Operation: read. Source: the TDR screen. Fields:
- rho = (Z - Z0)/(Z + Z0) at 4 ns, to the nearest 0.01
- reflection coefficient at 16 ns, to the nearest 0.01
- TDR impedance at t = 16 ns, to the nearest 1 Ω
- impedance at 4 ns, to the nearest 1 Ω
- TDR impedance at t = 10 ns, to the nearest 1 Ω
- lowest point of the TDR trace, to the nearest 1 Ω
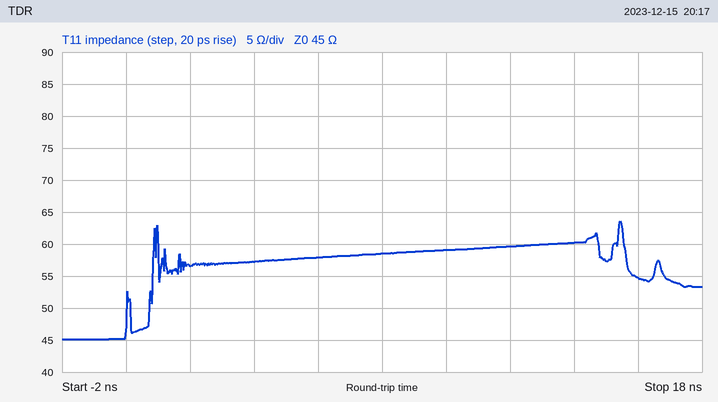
+0.12
+0.10
55 Ω
57 Ω
59 Ω
45 Ω
